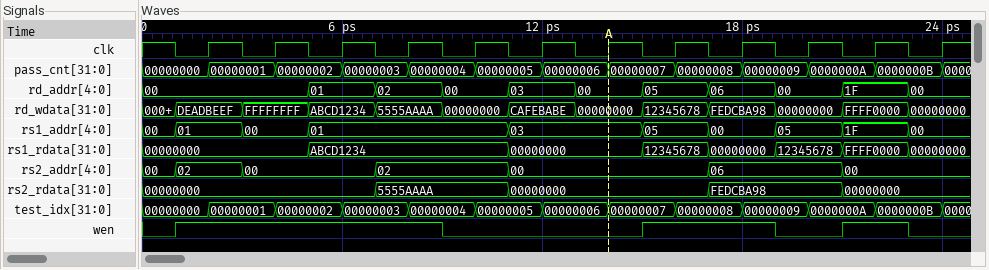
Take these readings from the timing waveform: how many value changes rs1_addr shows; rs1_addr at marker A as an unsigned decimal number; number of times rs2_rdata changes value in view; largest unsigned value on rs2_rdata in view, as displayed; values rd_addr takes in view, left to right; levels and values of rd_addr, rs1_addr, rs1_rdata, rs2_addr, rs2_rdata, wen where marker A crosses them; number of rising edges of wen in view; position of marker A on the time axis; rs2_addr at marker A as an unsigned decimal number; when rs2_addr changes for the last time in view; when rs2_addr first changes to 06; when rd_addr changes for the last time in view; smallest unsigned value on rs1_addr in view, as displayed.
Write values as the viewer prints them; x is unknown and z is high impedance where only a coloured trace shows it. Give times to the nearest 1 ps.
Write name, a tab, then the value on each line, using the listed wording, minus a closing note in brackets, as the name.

how many value changes rs1_addr shows	9
rs1_addr at marker A as an unsigned decimal number	3
number of times rs2_rdata changes value in view	4
largest unsigned value on rs2_rdata in view, as displayed	FEDCBA98
values rd_addr takes in view, left to right	00, 01, 02, 00, 03, 00, 05, 06, 00, 1F, 00
levels and values of rd_addr, rs1_addr, rs1_rdata, rs2_addr, rs2_rdata, wen where marker A crosses them	rd_addr=00, rs1_addr=03, rs1_rdata=00000000, rs2_addr=00, rs2_rdata=00000000, wen=0
number of rising edges of wen in view	3
position of marker A on the time axis	14 ps
rs2_addr at marker A as an unsigned decimal number	0
when rs2_addr changes for the last time in view	21 ps
when rs2_addr first changes to 06	17 ps
when rd_addr changes for the last time in view	23 ps
smallest unsigned value on rs1_addr in view, as displayed	00
